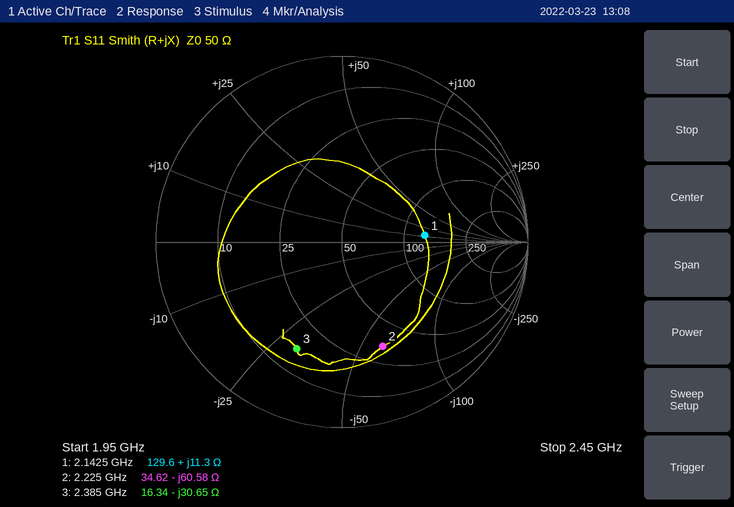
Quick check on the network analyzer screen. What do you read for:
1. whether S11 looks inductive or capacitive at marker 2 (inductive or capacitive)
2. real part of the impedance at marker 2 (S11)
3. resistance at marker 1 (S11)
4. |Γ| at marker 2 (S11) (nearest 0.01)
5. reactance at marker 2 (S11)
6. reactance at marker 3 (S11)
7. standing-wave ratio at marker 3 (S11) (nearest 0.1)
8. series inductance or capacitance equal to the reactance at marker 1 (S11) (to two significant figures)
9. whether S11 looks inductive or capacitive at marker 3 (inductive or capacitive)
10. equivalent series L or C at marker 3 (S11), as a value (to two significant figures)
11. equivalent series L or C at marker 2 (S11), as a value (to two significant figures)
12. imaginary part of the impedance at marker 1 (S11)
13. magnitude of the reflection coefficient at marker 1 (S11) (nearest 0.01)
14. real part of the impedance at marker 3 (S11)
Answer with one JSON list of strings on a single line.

["capacitive", "34.62 Ω", "129.6 Ω", "0.60", "-60.58 Ω", "-30.65 Ω", "4.3", "840 pH", "capacitive", "2.2 pF", "1.2 pF", "+11.3 Ω", "0.45", "16.34 Ω"]
